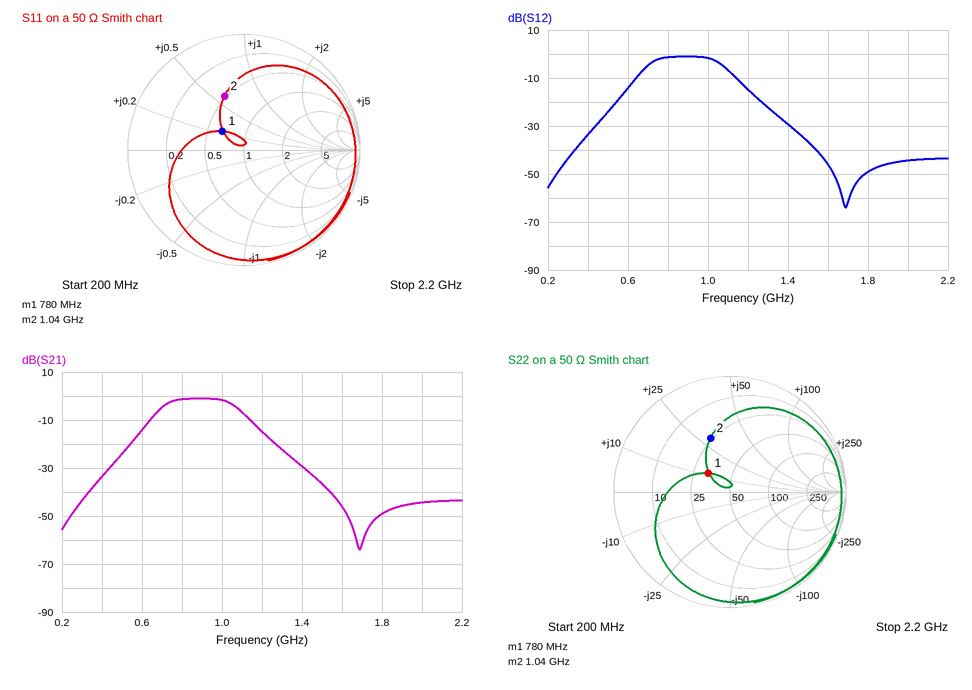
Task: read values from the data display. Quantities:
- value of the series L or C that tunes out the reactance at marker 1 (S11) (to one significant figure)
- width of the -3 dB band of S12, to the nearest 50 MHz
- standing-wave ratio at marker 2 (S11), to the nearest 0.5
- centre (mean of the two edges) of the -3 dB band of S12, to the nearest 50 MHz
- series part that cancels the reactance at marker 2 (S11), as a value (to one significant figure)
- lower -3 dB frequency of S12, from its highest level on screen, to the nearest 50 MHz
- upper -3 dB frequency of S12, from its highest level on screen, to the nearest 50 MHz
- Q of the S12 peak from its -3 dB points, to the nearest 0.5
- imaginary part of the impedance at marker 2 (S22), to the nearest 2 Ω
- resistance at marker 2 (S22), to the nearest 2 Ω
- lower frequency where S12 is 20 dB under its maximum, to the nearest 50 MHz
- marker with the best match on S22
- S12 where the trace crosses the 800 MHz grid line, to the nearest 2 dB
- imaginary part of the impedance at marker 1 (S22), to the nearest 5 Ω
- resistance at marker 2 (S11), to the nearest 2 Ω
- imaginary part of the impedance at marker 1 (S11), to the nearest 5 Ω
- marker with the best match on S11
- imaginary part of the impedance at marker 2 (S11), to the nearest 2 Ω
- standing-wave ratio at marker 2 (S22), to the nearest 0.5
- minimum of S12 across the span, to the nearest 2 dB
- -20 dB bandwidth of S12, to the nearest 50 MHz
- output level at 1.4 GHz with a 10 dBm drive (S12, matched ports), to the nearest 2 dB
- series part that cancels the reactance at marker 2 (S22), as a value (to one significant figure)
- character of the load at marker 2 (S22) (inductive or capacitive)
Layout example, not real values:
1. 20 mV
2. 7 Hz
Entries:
1. 20 pF
2. 350 MHz
3. 3.0
4. 900 MHz
5. 5 pF
6. 700 MHz
7. 1.05 GHz
8. 2.5
9. +30 Ω
10. 24 Ω
11. 550 MHz
12. marker 1
13. -2 dB
14. +10 Ω
15. 24 Ω
16. +10 Ω
17. marker 1
18. +30 Ω
19. 3.0
20. -64 dB
21. 750 MHz
22. -20 dBm
23. 5 pF
24. inductive
